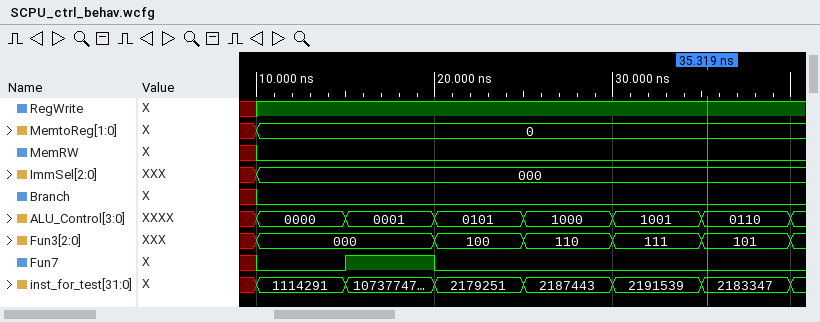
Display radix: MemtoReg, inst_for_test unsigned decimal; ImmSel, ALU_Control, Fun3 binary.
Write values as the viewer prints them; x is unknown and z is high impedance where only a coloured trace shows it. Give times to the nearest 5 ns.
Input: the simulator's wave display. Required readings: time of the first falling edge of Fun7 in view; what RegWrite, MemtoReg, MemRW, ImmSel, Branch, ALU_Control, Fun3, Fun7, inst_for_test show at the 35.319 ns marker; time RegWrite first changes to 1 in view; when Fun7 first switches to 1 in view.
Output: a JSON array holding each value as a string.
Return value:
["20 ns", "RegWrite=1, MemtoReg=0, MemRW=0, ImmSel=000, Branch=0, ALU_Control=0110, Fun3=101, Fun7=0, inst_for_test=2183347", "10 ns", "15 ns"]
